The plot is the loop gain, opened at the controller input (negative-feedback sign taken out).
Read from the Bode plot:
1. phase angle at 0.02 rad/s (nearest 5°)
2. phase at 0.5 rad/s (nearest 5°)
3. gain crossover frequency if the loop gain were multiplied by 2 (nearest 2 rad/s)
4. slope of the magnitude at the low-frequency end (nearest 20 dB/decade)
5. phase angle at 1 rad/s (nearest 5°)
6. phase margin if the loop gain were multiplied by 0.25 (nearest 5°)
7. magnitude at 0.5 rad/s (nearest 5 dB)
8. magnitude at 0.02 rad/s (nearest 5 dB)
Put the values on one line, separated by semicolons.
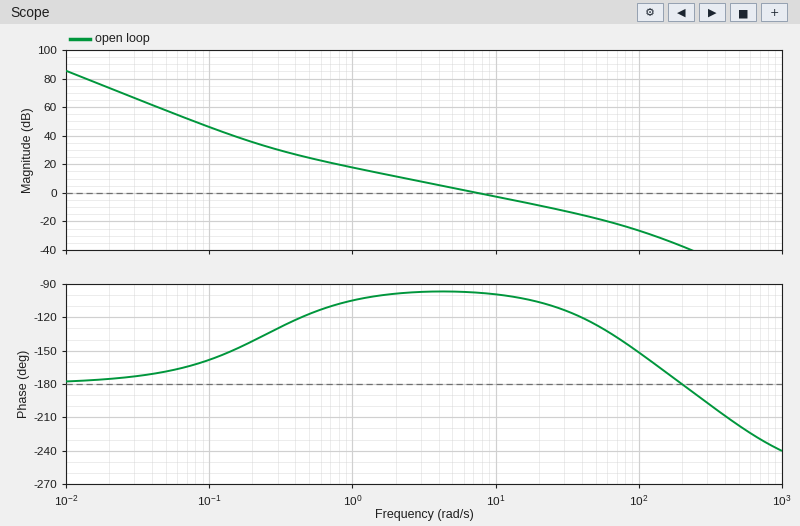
-175°; -115°; 14 rad/s; -40 dB/decade; -105°; 80°; 25 dB; 75 dB
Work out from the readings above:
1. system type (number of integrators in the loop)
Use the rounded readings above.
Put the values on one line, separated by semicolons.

2
